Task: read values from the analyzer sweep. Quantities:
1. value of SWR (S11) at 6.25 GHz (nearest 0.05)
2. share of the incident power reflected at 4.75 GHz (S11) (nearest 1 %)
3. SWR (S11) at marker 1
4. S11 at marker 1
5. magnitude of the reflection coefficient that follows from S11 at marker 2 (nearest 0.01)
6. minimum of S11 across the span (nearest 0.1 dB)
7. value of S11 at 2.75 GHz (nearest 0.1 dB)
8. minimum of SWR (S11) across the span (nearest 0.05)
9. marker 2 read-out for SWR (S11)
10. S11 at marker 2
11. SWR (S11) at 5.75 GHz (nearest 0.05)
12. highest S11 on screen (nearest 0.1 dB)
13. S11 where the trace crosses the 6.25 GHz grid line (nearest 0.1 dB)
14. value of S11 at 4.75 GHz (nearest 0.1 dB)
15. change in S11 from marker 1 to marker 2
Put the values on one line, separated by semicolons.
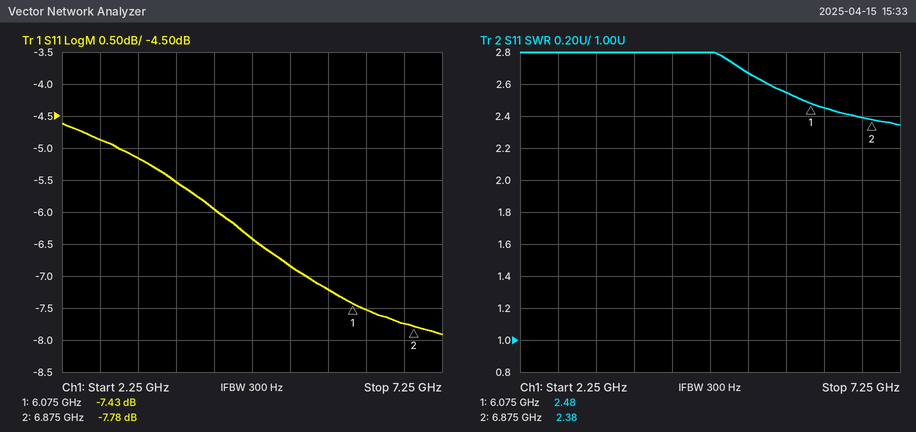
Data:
2.45; 23 %; 2.48; -7.43 dB; 0.41; -7.9 dB; -4.9 dB; 2.35; 2.38; -7.78 dB; 2.55; -4.6 dB; -7.5 dB; -6.4 dB; -0.35 dB
